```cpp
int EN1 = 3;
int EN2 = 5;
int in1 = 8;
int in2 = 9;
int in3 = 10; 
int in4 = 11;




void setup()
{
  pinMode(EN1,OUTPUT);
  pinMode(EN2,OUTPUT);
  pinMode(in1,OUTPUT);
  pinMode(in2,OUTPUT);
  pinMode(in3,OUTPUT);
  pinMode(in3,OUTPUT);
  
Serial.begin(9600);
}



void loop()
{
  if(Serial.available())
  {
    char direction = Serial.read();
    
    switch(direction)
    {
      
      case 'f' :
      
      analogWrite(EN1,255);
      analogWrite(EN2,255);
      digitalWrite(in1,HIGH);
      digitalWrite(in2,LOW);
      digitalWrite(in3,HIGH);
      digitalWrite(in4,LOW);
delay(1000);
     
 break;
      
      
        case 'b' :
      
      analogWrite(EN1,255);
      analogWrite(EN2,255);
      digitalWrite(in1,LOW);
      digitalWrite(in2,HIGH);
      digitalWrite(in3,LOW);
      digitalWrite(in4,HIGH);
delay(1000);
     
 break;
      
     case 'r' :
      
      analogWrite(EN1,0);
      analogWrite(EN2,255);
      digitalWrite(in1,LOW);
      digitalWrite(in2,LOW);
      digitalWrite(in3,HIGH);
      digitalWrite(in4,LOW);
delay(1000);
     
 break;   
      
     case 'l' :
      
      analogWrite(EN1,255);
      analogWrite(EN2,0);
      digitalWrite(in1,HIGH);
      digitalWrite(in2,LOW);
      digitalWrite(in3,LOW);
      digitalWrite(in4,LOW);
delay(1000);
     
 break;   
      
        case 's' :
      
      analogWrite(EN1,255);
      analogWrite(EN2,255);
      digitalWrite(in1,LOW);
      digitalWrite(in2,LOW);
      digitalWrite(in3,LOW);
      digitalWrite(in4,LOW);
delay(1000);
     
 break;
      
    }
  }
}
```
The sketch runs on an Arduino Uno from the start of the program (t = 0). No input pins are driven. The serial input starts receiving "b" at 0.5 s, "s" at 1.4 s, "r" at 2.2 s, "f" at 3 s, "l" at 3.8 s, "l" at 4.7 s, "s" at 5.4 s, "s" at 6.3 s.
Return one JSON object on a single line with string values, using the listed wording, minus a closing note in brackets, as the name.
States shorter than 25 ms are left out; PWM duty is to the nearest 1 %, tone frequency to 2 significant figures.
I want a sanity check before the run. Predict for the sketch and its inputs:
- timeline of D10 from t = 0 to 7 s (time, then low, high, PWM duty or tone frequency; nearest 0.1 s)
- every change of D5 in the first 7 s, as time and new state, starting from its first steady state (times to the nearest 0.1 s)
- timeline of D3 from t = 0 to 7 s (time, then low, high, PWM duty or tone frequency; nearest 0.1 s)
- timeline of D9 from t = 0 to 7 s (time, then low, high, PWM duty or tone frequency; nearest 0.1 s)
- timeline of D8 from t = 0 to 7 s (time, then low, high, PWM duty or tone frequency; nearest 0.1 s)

{"timeline of D10 from t = 0 to 7 s": "0 s low; 2.5 s high; 4.5 s low", "every change of D5 in the first 7 s, as time and new state, starting from its first steady state": "0 s low; 0.5 s high; 4.5 s low; 6.5 s high", "timeline of D3 from t = 0 to 7 s": "0 s low; 0.5 s high; 2.5 s low; 3.5 s high", "timeline of D9 from t = 0 to 7 s": "0 s low; 0.5 s high; 1.5 s low", "timeline of D8 from t = 0 to 7 s": "0 s low; 3.5 s high; 6.5 s low"}
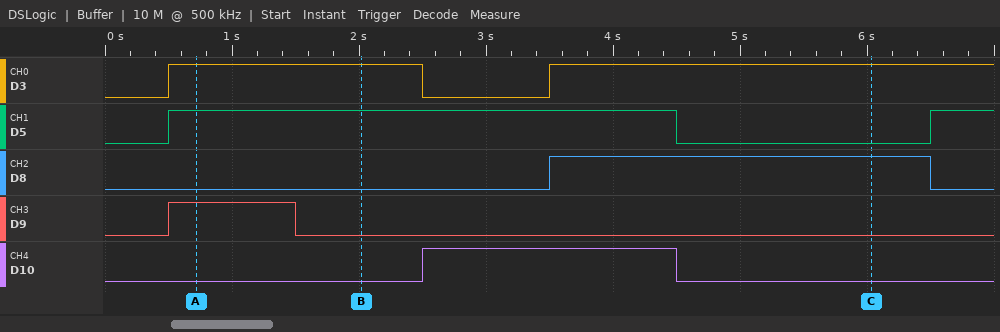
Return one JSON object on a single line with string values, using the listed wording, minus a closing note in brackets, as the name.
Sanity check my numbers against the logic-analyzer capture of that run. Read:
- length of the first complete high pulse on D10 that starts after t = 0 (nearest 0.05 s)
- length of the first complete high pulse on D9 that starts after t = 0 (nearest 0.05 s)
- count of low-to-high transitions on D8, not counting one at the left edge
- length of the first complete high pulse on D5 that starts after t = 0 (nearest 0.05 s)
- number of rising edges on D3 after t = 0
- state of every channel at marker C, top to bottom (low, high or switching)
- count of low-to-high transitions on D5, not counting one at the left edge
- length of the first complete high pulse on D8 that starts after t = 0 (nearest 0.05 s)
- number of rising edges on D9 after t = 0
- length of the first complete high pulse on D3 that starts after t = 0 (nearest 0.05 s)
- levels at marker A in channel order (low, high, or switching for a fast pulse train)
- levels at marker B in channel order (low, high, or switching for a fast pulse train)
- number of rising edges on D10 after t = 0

{"length of the first complete high pulse on D10 that starts after t = 0": "2.00 s", "length of the first complete high pulse on D9 that starts after t = 0": "1.00 s", "count of low-to-high transitions on D8, not counting one at the left edge": "1", "length of the first complete high pulse on D5 that starts after t = 0": "4.00 s", "number of rising edges on D3 after t = 0": "2", "state of every channel at marker C, top to bottom": "D3 high, D5 low, D8 high, D9 low, D10 low", "count of low-to-high transitions on D5, not counting one at the left edge": "2", "length of the first complete high pulse on D8 that starts after t = 0": "3.00 s", "number of rising edges on D9 after t = 0": "1", "length of the first complete high pulse on D3 that starts after t = 0": "2.00 s", "levels at marker A in channel order": "D3 high, D5 high, D8 low, D9 high, D10 low", "levels at marker B in channel order": "D3 high, D5 high, D8 low, D9 low, D10 low", "number of rising edges on D10 after t = 0": "1"}
